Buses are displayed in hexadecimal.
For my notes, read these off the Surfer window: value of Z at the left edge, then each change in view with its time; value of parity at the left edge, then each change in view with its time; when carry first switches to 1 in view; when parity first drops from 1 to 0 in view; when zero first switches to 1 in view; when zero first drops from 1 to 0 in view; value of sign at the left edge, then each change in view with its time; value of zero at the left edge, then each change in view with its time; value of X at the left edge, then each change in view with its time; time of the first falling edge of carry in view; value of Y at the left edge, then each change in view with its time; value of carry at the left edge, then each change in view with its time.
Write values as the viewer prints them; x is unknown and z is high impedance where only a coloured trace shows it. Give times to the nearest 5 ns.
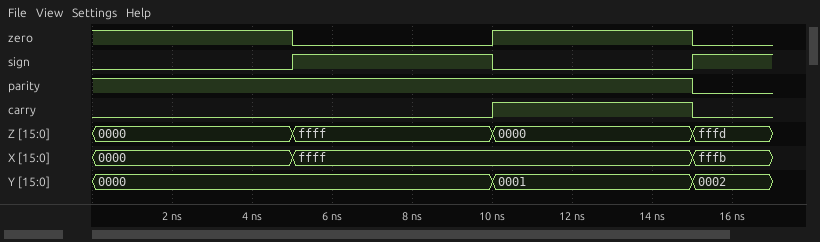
0000, ffff at 5 ns, 0000 at 10 ns, fffd at 15 ns
1, 0 at 15 ns
10 ns
15 ns
10 ns
5 ns
0, 1 at 5 ns, 0 at 10 ns, 1 at 15 ns
1, 0 at 5 ns, 1 at 10 ns, 0 at 15 ns
0000, ffff at 5 ns, fffb at 15 ns
15 ns
0000, 0001 at 10 ns, 0002 at 15 ns
0, 1 at 10 ns, 0 at 15 ns
